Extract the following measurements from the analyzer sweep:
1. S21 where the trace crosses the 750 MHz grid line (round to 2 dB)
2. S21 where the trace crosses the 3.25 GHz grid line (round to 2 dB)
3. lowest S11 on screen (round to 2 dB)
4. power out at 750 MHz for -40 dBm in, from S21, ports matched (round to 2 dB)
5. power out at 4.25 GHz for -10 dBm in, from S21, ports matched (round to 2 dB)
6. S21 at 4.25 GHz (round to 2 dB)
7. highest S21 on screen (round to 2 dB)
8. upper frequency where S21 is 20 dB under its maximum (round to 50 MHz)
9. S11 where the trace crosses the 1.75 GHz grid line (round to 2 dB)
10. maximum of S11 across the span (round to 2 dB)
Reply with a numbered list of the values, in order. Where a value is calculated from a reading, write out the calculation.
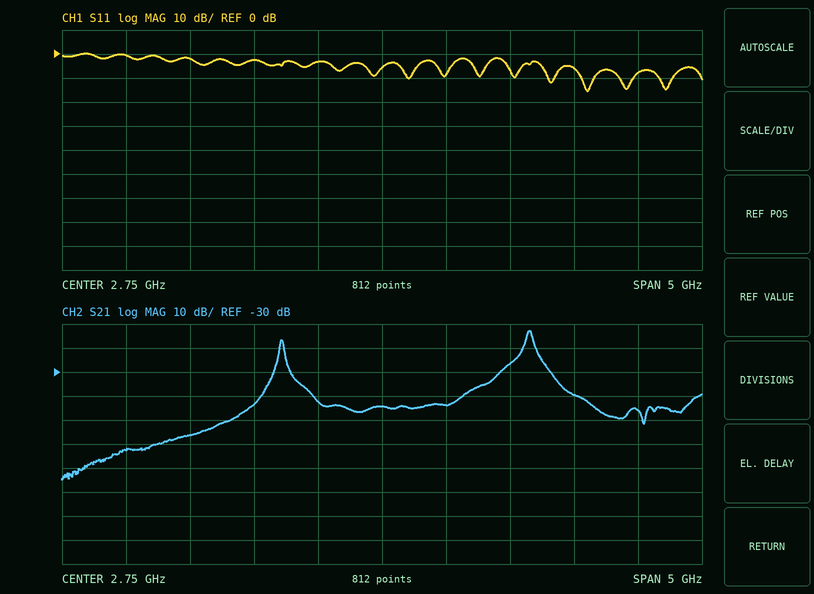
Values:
1. -62 dB
2. -44 dB
3. -16 dB
4. -40 dBm + (-62 dB) = -102 dBm
5. -10 dBm + (-40 dB) = -50 dBm
6. -40 dB
7. -12 dB
8. 4.10 GHz
9. -2 dB
10. 0 dB
